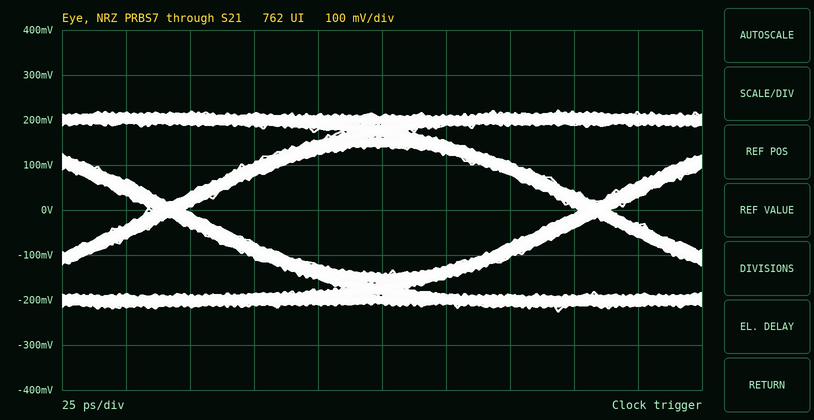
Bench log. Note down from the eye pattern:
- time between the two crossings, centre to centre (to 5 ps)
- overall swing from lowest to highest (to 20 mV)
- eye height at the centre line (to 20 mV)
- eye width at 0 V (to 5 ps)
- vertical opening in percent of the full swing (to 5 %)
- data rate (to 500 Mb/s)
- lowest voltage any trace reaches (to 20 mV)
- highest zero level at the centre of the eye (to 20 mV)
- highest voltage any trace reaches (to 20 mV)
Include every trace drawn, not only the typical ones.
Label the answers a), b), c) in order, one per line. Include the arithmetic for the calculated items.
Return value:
a) 165 ps
b) 440 mV
c) 280 mV
d) 155 ps
e) 280 mV / 440 mV ≈ 63.6 %, so 65 % to the nearest 5 %
f) 6.0 Gb/s
g) -220 mV
h) -140 mV
i) 220 mV
